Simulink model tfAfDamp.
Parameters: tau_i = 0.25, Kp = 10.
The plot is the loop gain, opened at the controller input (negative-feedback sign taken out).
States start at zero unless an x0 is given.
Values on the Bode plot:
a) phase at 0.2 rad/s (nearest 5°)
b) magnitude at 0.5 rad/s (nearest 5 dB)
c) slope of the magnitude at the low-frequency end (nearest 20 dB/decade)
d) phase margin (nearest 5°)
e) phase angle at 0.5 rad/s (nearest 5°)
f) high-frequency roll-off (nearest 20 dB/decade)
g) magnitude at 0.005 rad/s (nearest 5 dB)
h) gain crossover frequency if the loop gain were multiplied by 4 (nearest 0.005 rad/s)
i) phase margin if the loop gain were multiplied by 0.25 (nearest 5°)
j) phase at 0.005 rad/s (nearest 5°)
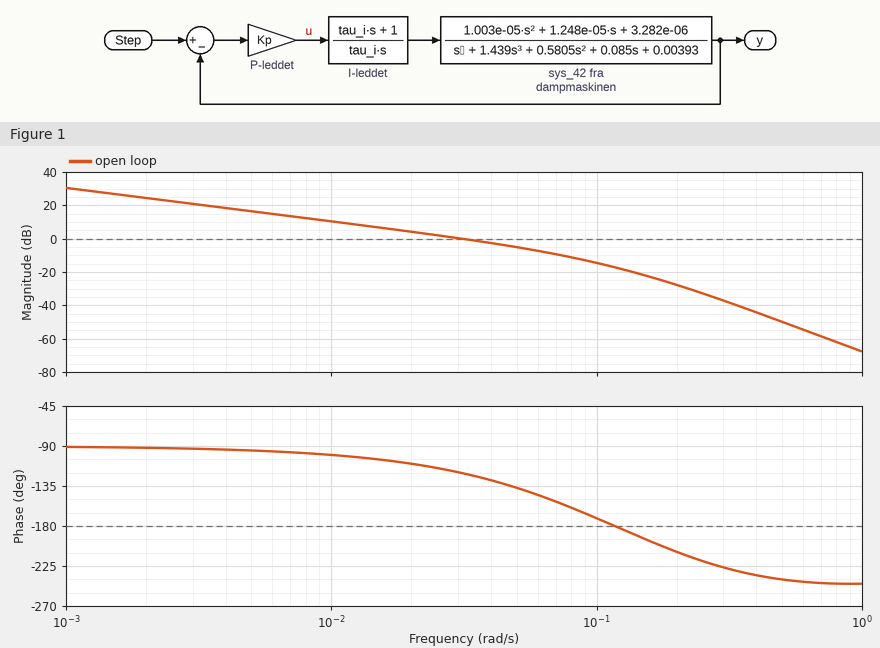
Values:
-210°
-50 dB
-20 dB/decade
60°
-240°
-60 dB/decade
15 dB
0.085 rad/s
80°
-95°
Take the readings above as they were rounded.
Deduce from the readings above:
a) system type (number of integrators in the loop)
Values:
1
